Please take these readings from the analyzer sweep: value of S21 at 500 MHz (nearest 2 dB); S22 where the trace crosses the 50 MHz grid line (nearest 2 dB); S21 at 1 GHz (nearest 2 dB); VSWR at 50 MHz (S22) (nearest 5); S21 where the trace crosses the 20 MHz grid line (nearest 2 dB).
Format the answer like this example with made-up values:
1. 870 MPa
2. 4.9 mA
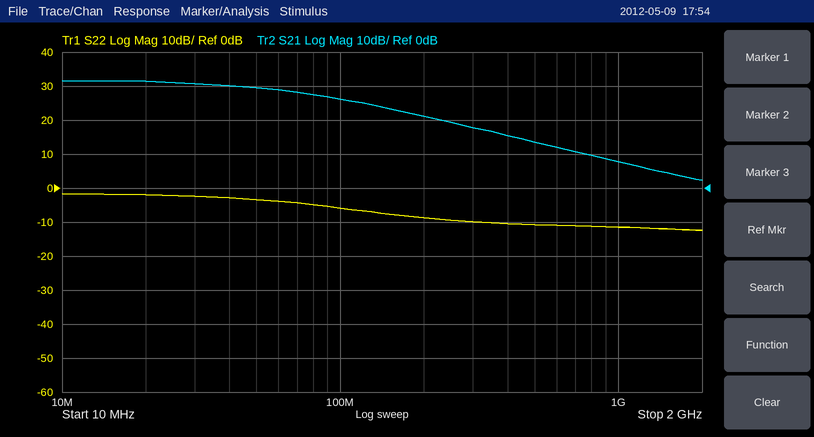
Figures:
1. 14 dB
2. -4 dB
3. 8 dB
4. 5
5. 32 dB
